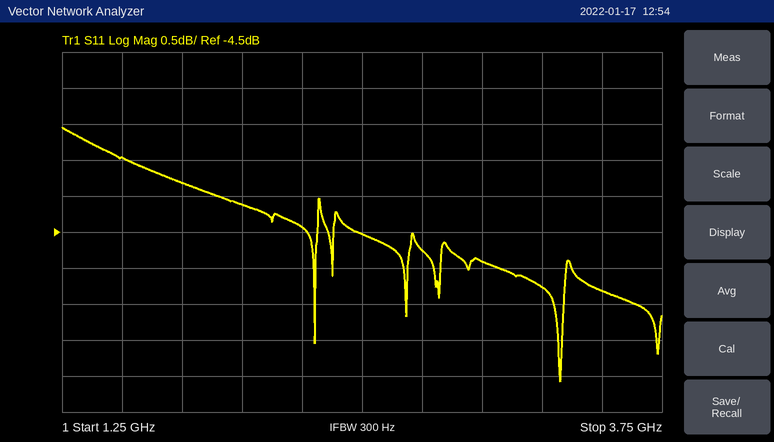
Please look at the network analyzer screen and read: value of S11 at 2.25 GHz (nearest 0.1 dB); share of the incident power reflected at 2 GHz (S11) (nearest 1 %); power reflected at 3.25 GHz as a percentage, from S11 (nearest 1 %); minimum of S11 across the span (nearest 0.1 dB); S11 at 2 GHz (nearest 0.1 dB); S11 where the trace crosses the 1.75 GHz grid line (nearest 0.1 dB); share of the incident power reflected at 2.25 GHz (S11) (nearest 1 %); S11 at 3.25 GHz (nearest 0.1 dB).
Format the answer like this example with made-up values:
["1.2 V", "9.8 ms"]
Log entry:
["-4.4 dB", "39 %", "30 %", "-6.6 dB", "-4.1 dB", "-3.8 dB", "36 %", "-5.3 dB"]
